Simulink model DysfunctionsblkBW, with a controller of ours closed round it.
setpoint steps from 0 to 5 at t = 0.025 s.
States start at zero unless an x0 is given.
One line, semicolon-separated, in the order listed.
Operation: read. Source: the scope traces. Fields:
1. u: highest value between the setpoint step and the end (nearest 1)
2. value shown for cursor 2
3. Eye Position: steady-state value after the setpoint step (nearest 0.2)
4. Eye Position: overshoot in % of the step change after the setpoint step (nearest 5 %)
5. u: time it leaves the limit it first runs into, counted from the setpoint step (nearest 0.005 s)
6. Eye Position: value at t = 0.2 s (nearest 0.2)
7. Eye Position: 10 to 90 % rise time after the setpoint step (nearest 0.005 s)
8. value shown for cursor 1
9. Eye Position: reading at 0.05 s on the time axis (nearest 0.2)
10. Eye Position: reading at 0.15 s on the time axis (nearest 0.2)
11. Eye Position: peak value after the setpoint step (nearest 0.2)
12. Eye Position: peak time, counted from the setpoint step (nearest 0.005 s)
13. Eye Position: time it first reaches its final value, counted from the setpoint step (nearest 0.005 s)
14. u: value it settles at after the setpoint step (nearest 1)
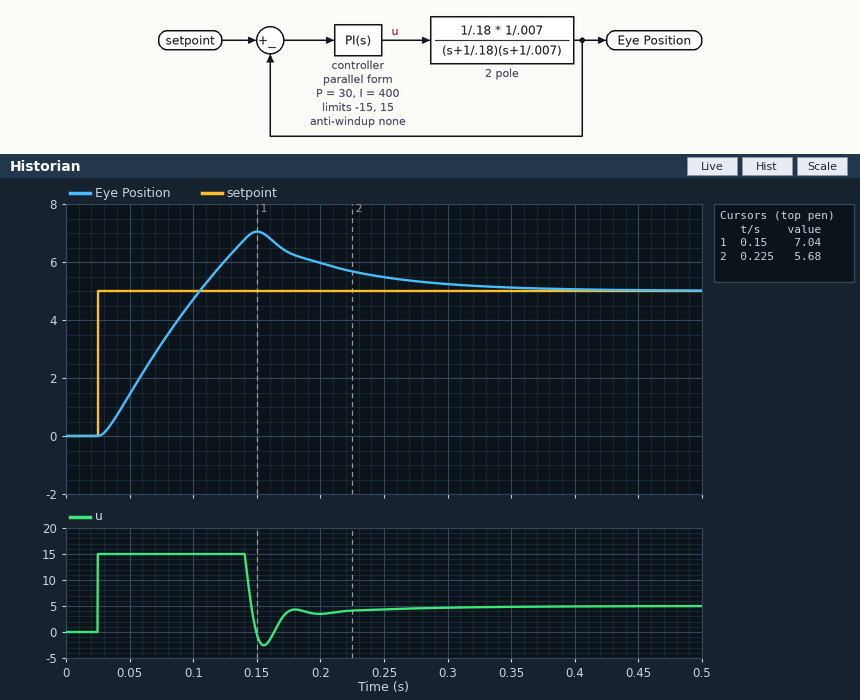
15; 5.68; 5.0; 40 %; 0.115 s; 6.0; 0.060 s; 7.04; 1.4; 7.0; 7.0; 0.125 s; 0.080 s; 5
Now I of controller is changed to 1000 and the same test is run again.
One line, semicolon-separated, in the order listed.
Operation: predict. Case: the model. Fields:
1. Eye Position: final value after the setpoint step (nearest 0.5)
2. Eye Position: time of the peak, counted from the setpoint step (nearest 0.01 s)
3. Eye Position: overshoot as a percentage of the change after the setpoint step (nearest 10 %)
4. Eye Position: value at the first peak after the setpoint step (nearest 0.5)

5.0; 0.15 s; 60 %; 8.0
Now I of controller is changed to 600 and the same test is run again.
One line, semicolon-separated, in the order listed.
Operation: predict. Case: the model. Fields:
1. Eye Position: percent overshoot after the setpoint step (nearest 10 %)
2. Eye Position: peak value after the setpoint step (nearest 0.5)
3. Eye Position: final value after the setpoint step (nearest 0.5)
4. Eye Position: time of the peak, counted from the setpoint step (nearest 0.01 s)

50 %; 7.5; 5.0; 0.14 s
